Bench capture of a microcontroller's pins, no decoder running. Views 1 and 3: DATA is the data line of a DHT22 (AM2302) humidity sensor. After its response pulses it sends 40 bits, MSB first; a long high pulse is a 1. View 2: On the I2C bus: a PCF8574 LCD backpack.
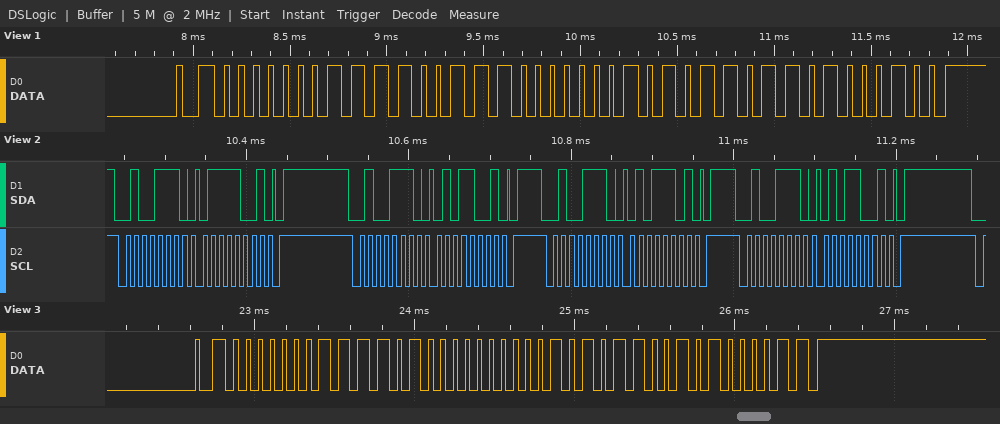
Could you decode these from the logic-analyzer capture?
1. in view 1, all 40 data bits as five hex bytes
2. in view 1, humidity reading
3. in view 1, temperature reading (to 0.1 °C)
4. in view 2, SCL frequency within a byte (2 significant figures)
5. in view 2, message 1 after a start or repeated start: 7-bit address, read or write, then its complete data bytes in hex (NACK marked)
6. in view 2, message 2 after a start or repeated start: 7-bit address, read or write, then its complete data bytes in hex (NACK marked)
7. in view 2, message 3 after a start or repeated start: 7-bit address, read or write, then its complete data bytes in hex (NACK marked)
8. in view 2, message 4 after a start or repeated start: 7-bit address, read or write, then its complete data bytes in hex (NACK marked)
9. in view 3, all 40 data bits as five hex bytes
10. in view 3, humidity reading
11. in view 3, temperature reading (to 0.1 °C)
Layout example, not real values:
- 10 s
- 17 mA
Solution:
- 01 E7 01 5B 44
- 48.7 %
- 34.7 °C
- 100 kHz
- 0x27 write: 79
- 0x27 write: 59
- 0x27 write: 5D
- 0x27 write: 59
- 01 E8 01 59 43
- 48.8 %
- 34.5 °C
